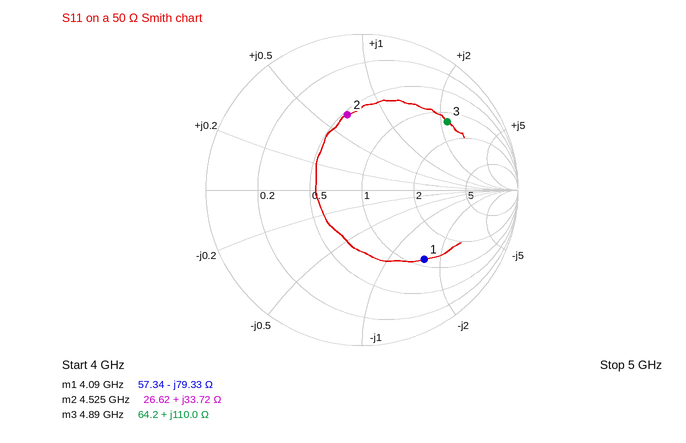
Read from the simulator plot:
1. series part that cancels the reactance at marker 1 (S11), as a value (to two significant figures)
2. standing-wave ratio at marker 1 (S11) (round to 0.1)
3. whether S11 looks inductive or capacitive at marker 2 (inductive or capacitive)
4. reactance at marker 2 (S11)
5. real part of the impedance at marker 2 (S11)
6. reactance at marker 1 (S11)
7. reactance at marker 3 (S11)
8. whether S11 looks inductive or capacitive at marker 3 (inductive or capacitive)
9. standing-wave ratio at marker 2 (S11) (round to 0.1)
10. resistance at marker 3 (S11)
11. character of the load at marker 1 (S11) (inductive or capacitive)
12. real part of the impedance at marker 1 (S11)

3.1 nH
4.0
inductive
+33.72 Ω
26.62 Ω
-79.33 Ω
+110.0 Ω
inductive
2.9
64.2 Ω
capacitive
57.34 Ω
